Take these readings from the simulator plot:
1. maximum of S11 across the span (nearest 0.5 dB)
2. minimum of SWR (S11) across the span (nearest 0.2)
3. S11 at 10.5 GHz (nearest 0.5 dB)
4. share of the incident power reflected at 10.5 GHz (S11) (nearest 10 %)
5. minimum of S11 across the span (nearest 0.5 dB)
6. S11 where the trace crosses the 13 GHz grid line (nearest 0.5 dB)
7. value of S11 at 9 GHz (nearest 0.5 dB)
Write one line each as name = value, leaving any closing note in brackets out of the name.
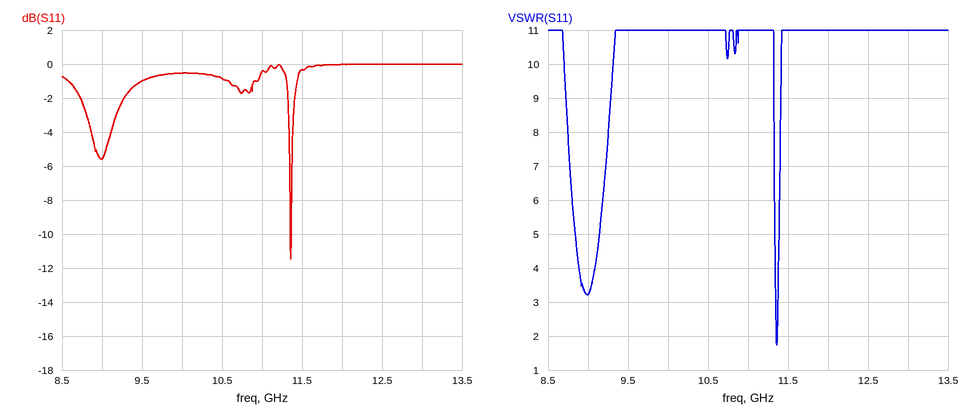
maximum of S11 across the span = 0.0 dB
minimum of SWR (S11) across the span = 1.8
S11 at 10.5 GHz = -1.0 dB
share of the incident power reflected at 10.5 GHz (S11) = 80 %
minimum of S11 across the span = -11.5 dB
S11 where the trace crosses the 13 GHz grid line = 0.0 dB
value of S11 at 9 GHz = -5.5 dB
